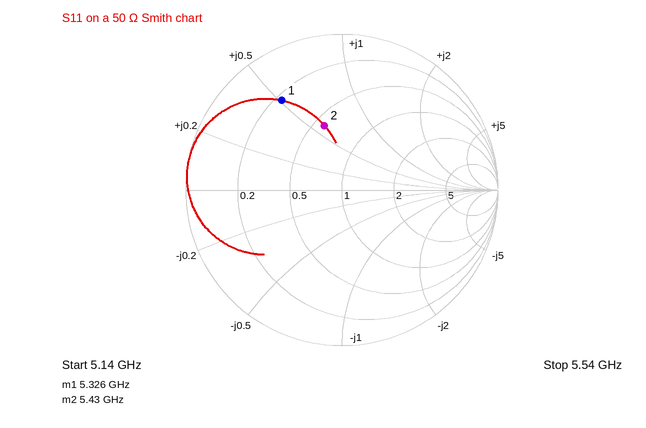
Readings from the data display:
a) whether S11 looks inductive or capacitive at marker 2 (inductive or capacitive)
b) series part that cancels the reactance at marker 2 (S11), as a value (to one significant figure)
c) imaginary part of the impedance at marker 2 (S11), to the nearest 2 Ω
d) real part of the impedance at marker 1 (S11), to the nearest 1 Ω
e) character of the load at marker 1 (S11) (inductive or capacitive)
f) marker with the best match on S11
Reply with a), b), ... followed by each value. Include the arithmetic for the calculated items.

a) inductive
b) C = 1/(2π × 5.43 GHz × 30 Ω) ≈ 1.0 pF
c) +30 Ω
d) 12 Ω
e) inductive
f) marker 2
